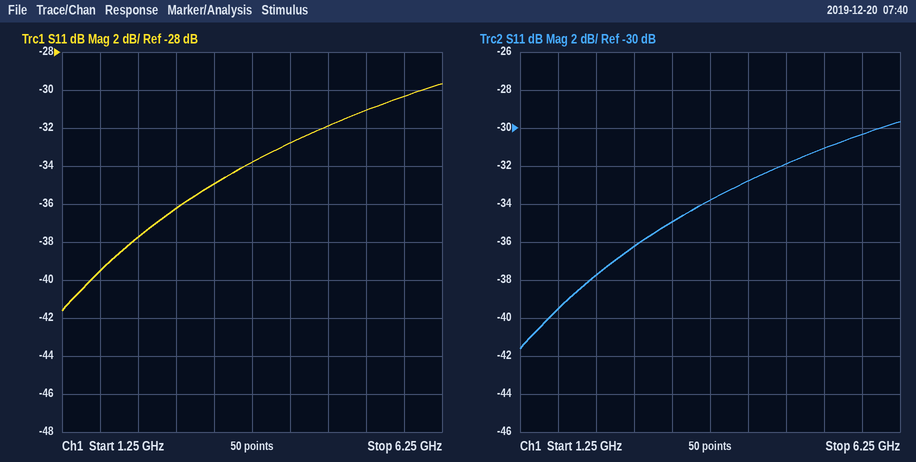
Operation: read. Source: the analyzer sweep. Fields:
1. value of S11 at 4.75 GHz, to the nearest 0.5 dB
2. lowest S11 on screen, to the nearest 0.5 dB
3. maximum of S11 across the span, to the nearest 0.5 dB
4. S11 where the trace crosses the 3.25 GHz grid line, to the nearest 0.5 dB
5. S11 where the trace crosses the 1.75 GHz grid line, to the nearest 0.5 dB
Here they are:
-32.0 dB
-41.5 dB
-29.5 dB
-35.0 dB
-39.5 dB
